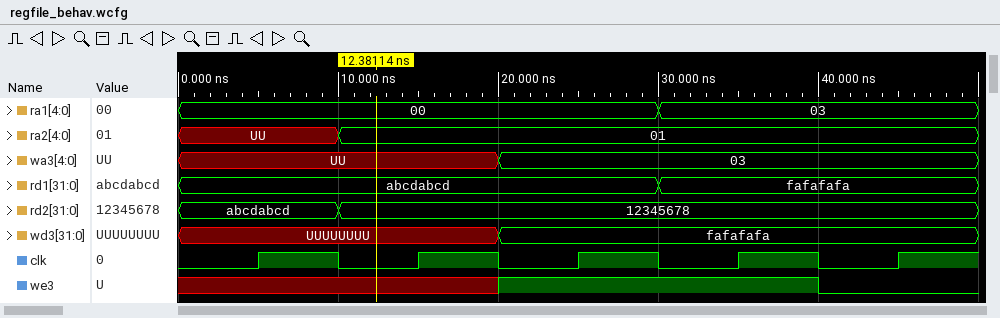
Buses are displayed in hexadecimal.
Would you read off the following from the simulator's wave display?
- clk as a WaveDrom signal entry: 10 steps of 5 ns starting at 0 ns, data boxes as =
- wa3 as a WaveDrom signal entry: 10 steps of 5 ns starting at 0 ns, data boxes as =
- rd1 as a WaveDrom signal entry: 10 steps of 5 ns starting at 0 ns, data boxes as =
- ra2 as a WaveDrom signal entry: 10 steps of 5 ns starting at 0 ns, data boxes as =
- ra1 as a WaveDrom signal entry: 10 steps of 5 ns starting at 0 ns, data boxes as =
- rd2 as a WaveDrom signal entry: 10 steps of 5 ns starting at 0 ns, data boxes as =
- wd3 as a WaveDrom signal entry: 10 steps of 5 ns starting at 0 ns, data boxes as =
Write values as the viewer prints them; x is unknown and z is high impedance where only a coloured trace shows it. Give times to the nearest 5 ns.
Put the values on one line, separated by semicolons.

{name: 'clk', wave: '0101010101'}; {name: 'wa3', wave: 'x...=.....', data: '03'}; {name: 'rd1', wave: '=.....=...', data: 'abcdabcd fafafafa'}; {name: 'ra2', wave: 'x.=.......', data: '01'}; {name: 'ra1', wave: '=.....=...', data: '00 03'}; {name: 'rd2', wave: '=.=.......', data: 'abcdabcd 12345678'}; {name: 'wd3', wave: 'x...=.....', data: 'fafafafa'}
